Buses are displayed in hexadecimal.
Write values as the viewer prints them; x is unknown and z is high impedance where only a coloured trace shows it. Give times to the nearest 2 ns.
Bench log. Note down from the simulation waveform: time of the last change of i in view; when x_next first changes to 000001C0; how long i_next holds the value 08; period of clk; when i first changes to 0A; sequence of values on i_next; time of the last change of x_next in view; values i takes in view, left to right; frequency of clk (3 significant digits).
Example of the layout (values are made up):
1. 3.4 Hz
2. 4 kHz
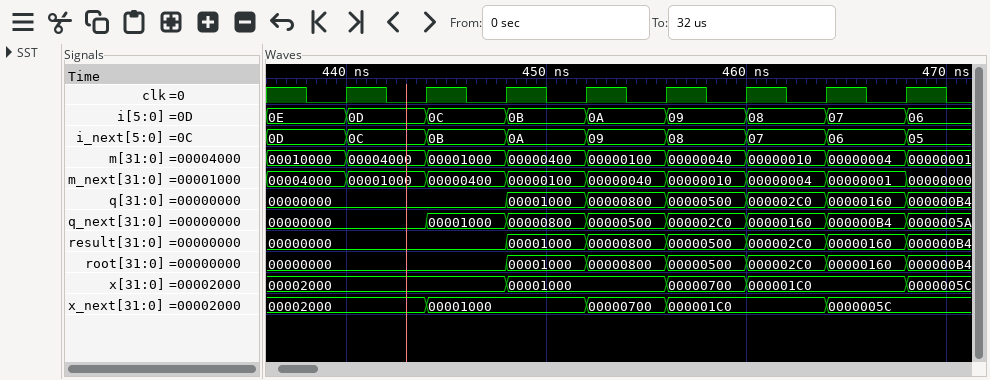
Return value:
1. 468 ns
2. 456 ns
3. 4 ns
4. 4 ns
5. 452 ns
6. 0D, 0C, 0B, 0A, 09, 08, 07, 06, 05
7. 464 ns
8. 0E, 0D, 0C, 0B, 0A, 09, 08, 07, 06
9. 250 MHz
